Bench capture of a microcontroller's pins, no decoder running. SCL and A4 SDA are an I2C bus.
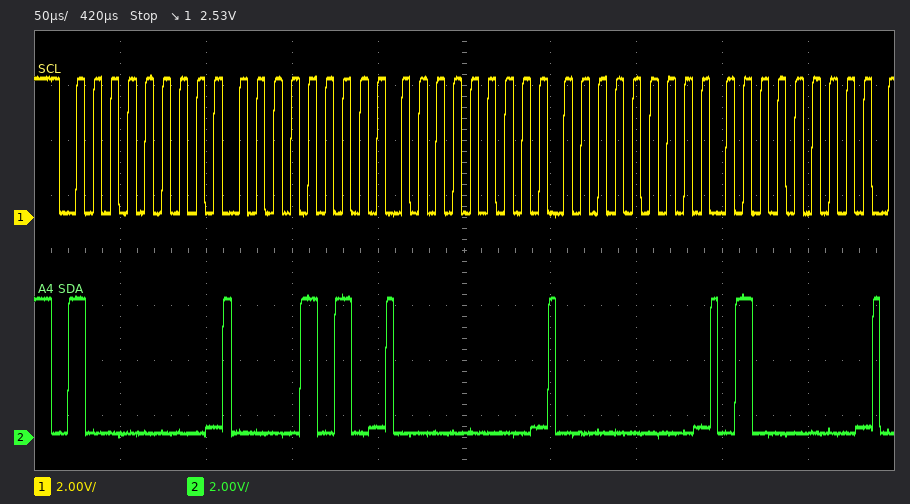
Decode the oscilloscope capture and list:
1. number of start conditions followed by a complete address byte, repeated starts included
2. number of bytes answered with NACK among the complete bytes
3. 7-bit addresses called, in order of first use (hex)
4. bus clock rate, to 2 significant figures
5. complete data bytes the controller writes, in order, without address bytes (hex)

1
0
0x40
100 kHz
0A 00 00 40
